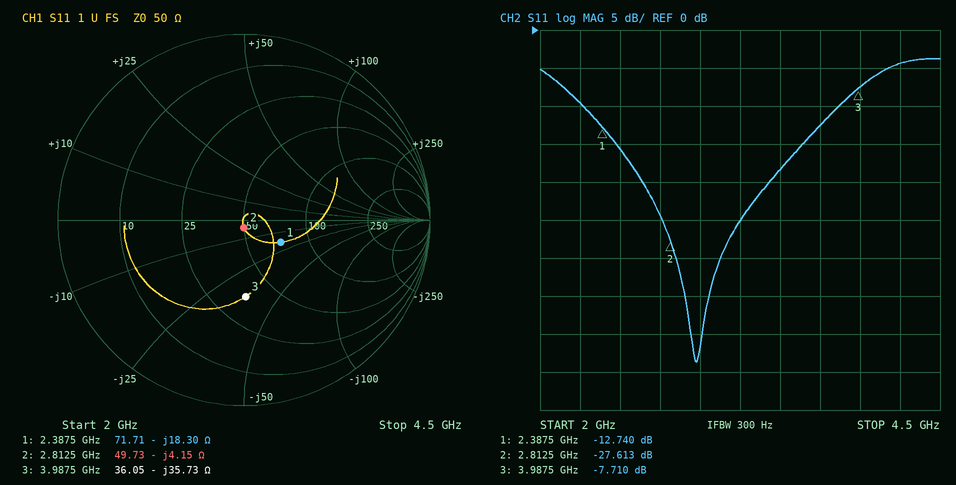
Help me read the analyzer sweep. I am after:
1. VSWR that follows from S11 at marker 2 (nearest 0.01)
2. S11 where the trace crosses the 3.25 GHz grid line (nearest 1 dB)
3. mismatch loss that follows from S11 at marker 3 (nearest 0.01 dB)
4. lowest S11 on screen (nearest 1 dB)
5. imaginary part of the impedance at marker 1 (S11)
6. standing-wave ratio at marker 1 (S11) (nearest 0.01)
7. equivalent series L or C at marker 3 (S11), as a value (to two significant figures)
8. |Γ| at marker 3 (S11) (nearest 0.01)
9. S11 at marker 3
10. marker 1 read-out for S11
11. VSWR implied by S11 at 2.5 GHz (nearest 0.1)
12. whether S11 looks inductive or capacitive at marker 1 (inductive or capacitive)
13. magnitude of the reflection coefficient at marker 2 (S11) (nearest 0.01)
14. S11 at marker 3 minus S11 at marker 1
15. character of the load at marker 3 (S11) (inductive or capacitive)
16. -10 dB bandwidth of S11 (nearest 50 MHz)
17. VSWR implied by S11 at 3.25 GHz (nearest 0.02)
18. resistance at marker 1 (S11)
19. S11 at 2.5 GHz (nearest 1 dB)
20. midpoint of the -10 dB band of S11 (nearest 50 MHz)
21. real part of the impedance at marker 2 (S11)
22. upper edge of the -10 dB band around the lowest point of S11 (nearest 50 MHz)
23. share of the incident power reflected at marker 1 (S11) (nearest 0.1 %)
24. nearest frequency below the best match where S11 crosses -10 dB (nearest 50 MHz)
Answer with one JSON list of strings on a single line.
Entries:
["1.09", "-25 dB", "0.81 dB", "-44 dB", "-18.30 Ω", "1.60", "1.1 pF", "0.41", "-7.710 dB", "-12.740 dB", "1.4", "capacitive", "0.04", "5.030 dB", "capacitive", "1.60 GHz", "1.12", "71.71 Ω", "-16 dB", "3.05 GHz", "49.73 Ω", "3.85 GHz", "5.3 %", "2.25 GHz"]
